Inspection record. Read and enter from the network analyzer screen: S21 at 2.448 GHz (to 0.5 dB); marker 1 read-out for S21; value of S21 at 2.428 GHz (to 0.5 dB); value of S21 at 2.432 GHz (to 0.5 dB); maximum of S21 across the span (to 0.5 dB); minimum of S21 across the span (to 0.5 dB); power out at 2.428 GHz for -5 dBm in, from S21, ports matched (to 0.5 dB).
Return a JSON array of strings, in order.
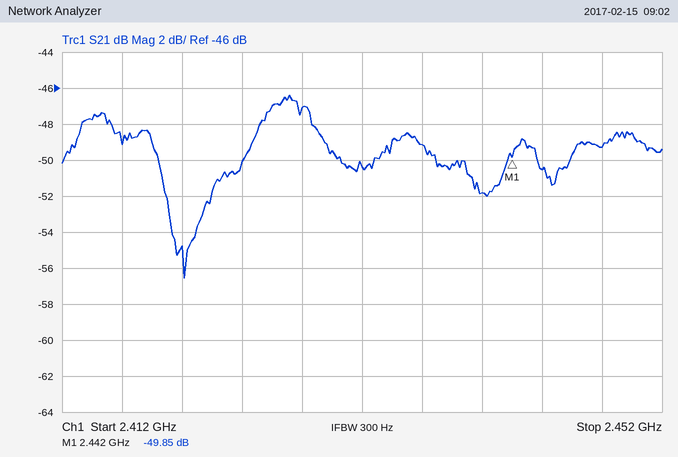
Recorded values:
["-49.5 dB", "-49.85 dB", "-47.0 dB", "-50.5 dB", "-46.5 dB", "-56.5 dB", "-52.0 dBm"]
